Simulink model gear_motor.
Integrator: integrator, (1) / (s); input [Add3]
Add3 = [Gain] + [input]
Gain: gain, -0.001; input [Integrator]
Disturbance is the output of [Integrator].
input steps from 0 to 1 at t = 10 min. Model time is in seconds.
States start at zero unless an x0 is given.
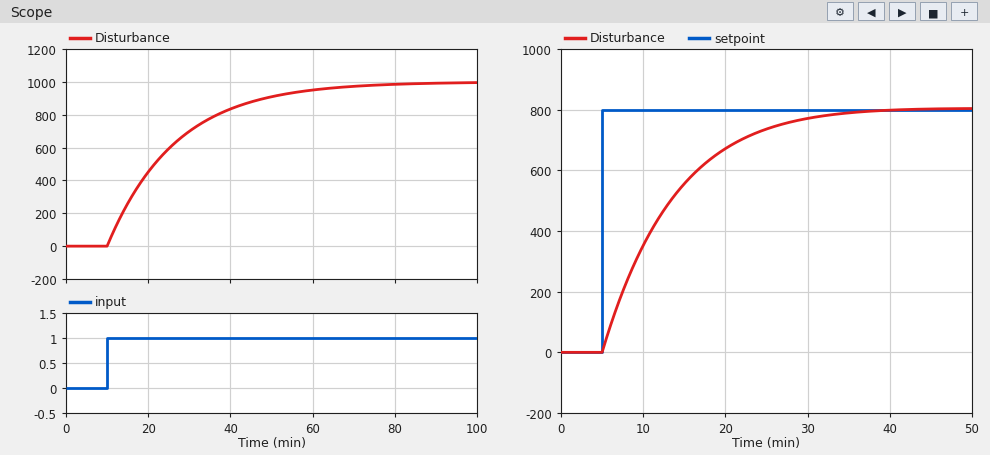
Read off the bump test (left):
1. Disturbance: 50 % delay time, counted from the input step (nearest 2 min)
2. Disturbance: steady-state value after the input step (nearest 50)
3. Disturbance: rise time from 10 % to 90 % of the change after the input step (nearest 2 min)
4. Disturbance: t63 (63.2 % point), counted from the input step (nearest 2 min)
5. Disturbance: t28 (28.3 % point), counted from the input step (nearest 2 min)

12 min
1000
36 min
16 min
6 min
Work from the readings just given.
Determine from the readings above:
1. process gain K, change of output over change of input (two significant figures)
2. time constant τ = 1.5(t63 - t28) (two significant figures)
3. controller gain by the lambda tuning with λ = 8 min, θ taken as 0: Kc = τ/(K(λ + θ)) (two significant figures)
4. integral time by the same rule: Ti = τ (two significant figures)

1000
15 min
0.0019
15 min
